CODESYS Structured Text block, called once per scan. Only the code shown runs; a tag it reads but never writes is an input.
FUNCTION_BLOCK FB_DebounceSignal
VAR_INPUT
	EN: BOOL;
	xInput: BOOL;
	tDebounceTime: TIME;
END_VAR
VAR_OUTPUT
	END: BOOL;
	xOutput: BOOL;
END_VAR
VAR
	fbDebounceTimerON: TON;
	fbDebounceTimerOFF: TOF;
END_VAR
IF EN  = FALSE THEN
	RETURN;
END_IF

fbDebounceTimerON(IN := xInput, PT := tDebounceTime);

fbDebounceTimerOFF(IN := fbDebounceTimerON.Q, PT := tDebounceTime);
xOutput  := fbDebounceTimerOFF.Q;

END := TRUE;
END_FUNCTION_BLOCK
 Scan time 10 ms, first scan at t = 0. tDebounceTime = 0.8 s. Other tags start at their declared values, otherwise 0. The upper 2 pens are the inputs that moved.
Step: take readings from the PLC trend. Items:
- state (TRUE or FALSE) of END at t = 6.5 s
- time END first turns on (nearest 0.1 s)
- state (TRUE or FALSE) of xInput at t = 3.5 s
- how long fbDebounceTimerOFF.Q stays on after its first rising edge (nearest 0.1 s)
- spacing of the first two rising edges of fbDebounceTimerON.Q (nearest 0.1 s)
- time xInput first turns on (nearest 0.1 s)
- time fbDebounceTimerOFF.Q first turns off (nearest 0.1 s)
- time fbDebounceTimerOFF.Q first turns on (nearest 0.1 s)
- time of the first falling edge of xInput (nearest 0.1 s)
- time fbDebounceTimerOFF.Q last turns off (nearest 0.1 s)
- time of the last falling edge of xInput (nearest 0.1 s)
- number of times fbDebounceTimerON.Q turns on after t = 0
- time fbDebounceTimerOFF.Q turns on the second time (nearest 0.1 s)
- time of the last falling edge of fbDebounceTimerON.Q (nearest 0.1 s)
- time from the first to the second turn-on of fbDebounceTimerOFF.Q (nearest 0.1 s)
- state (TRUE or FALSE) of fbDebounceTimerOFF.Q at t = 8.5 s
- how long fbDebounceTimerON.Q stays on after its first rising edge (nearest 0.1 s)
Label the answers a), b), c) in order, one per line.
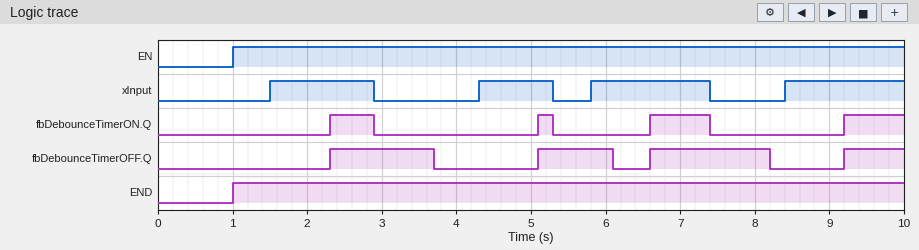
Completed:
a) TRUE
b) 1.0 s
c) FALSE
d) 1.4 s
e) 2.8 s
f) 1.5 s
g) 3.7 s
h) 2.3 s
i) 2.9 s
j) 8.2 s
k) 7.4 s
l) 4
m) 5.1 s
n) 7.4 s
o) 2.8 s
p) FALSE
q) 0.6 s
